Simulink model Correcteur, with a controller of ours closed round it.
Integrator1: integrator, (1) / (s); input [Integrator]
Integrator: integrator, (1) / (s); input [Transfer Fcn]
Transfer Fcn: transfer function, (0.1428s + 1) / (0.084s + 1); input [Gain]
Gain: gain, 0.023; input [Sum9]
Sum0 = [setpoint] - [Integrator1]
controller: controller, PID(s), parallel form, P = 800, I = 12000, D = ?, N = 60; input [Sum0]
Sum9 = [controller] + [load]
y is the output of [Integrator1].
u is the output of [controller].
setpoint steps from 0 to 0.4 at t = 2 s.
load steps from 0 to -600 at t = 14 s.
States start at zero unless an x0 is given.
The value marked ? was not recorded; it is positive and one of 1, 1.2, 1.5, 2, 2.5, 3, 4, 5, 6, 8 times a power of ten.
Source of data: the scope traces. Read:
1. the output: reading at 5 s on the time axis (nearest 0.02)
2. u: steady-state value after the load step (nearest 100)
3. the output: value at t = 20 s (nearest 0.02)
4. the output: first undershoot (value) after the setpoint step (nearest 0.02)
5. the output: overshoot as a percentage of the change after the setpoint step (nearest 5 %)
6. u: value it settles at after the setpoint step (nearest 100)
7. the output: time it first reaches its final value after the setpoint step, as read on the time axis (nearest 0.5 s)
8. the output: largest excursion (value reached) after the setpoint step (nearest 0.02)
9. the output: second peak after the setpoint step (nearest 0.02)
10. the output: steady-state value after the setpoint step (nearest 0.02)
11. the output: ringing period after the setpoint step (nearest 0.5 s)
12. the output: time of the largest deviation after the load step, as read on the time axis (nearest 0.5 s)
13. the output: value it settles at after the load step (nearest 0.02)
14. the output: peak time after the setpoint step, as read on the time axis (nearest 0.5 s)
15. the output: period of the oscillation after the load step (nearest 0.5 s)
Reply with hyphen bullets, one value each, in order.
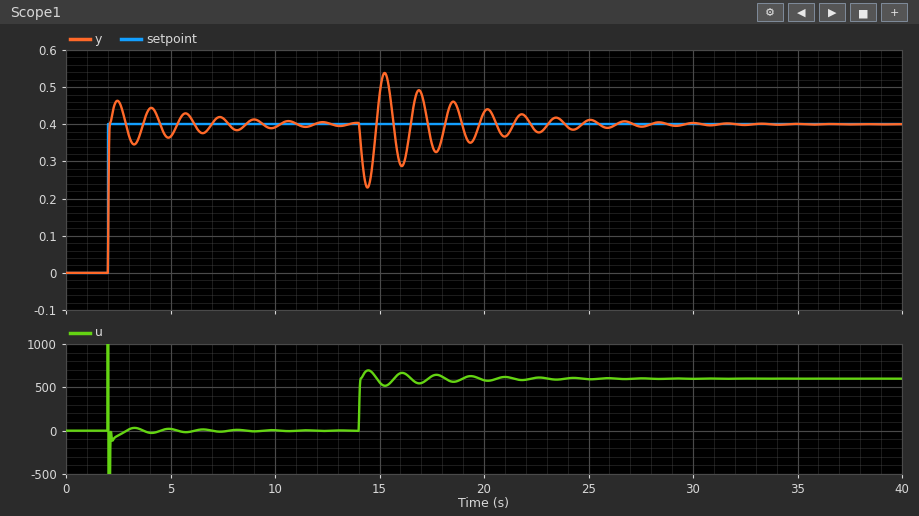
- 0.36
- 600
- 0.44
- 0.34
- 15 %
- 0
- 2.0 s
- 0.46
- 0.44
- 0.40
- 1.5 s
- 14.5 s
- 0.40
- 2.5 s
- 1.5 s
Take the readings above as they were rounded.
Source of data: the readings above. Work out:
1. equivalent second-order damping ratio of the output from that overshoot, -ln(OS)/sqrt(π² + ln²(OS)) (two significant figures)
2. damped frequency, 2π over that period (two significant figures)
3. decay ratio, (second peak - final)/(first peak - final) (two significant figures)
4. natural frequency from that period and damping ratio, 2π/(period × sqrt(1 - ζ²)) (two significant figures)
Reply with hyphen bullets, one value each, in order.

- 0.52
- 4.2 rad/s
- 0.67
- 4.9 rad/s
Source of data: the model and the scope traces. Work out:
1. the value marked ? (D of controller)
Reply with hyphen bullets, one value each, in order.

- 800
